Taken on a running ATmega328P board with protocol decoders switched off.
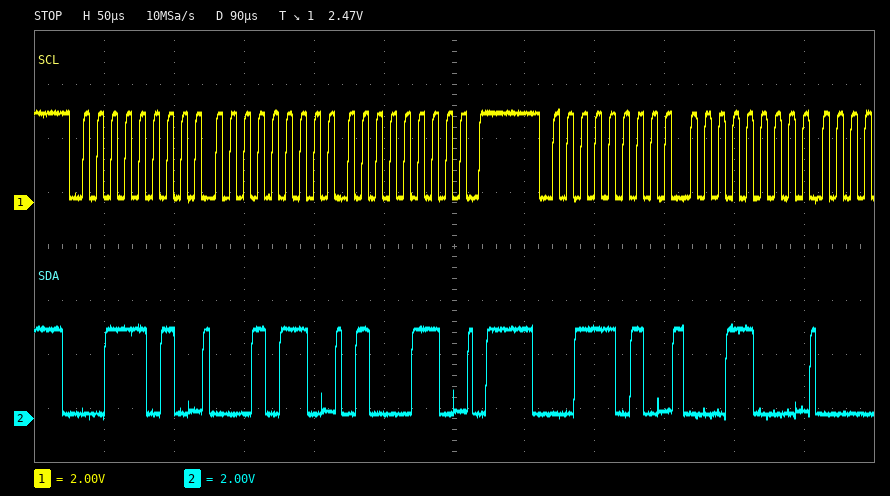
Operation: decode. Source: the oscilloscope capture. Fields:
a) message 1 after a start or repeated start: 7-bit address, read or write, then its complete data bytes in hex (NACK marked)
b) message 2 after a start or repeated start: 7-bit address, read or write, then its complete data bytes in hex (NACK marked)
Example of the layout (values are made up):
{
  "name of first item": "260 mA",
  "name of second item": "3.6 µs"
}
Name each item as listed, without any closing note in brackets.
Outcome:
{
  "message 1 after a start or repeated start: 7-bit address, read or write, then its complete data bytes in hex": "0x1D write: 16 46",
  "message 2 after a start or repeated start: 7-bit address, read or write, then its complete data bytes in hex": "0x1D write: 18"
}
